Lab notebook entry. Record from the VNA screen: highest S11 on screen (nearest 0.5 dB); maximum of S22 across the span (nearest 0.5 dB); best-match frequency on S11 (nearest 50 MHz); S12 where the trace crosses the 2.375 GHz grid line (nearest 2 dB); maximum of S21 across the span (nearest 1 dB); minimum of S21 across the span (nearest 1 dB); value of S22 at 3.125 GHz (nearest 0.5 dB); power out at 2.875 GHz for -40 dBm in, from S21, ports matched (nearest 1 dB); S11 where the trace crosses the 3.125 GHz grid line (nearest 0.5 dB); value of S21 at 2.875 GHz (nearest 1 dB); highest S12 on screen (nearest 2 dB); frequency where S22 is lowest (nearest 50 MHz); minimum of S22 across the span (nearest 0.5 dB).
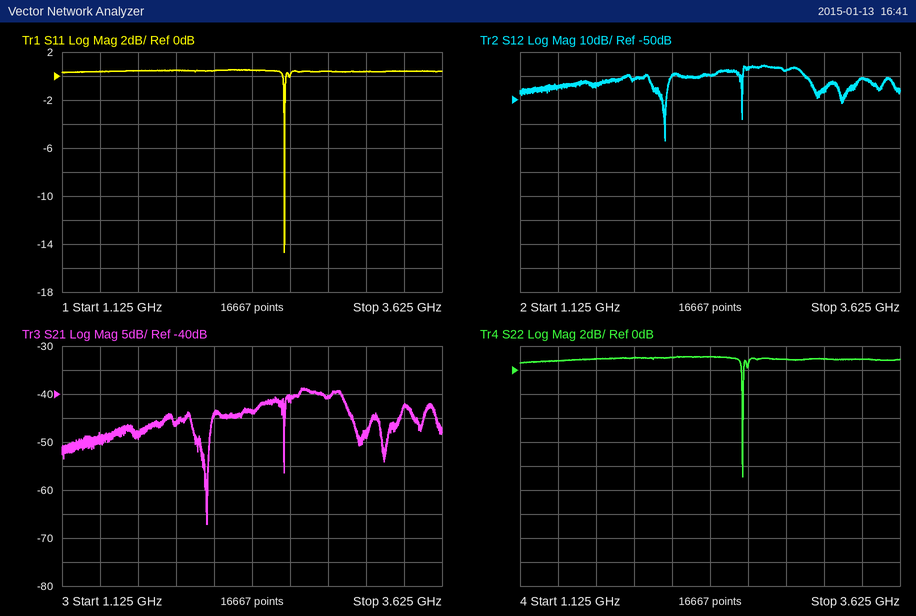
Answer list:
0.5 dB
1.0 dB
2.60 GHz
-40 dB
-39 dB
-67 dB
1.0 dB
-81 dBm
0.5 dB
-41 dB
-36 dB
2.60 GHz
-9.0 dB
